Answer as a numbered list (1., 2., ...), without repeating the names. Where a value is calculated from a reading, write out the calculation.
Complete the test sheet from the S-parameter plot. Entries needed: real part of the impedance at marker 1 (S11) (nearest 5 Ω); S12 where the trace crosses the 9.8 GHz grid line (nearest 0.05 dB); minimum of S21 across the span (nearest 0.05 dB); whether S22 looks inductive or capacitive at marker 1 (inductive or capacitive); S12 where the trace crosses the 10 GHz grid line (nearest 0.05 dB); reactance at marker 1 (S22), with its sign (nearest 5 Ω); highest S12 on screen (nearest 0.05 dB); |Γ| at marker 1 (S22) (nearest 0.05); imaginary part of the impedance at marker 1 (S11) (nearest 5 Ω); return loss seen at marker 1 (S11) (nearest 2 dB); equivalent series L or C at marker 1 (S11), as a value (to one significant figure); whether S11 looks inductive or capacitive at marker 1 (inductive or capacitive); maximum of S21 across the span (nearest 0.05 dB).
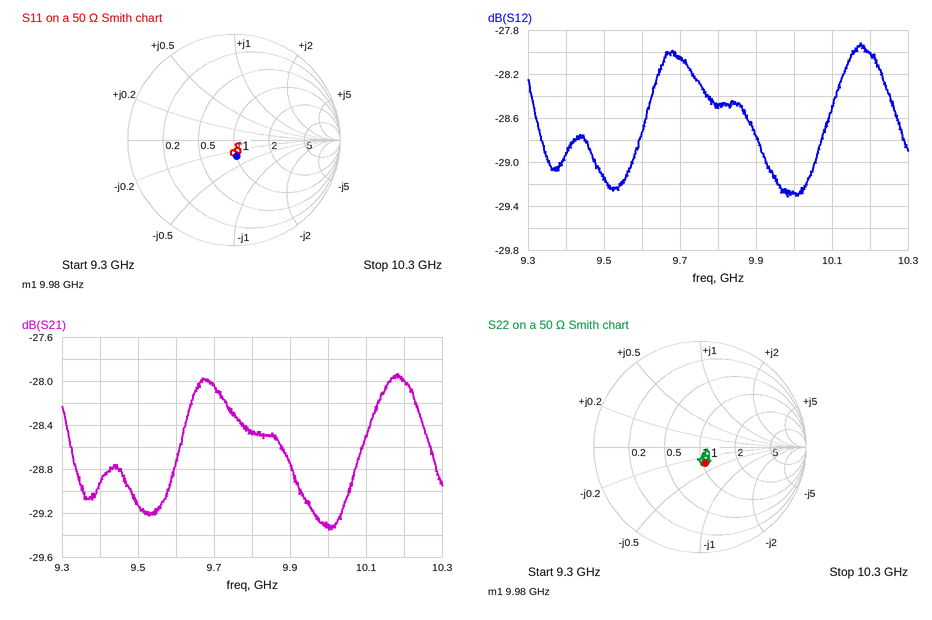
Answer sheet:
1. 50 Ω
2. -28.50 dB
3. -29.35 dB
4. capacitive
5. -29.30 dB
6. -15 Ω
7. -27.90 dB
8. 0.15
9. -15 Ω
10. 16 dB
11. C = 1/(2π × 9.98 GHz × 15 Ω) ≈ 1 pF
12. capacitive
13. -27.95 dB
